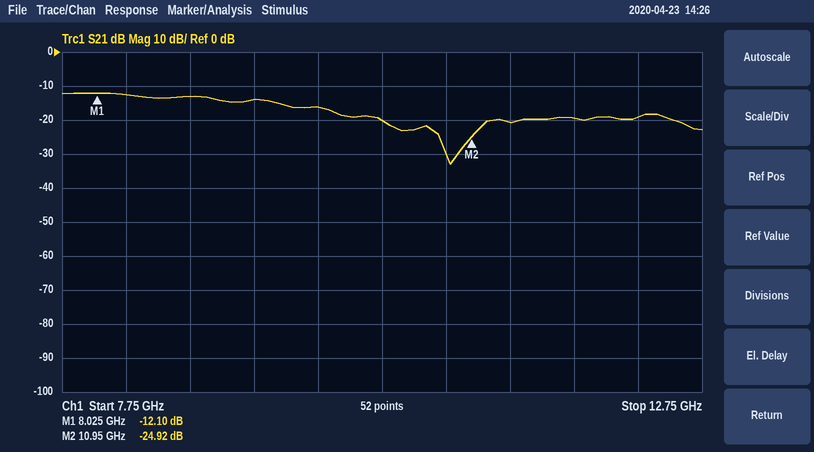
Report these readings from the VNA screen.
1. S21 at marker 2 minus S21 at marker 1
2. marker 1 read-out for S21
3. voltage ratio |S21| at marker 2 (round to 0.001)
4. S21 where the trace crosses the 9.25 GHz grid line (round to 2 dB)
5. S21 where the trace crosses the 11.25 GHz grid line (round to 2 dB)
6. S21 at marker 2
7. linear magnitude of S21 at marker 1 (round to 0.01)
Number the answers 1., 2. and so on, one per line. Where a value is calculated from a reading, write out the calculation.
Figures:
1. -24.92 − (-12.1) = -12.82 dB
2. -12.10 dB
3. 10^(-24.92/20) ≈ 0.057
4. -14 dB
5. -20 dB
6. -24.92 dB
7. 10^(-12.1/20) ≈ 0.25
